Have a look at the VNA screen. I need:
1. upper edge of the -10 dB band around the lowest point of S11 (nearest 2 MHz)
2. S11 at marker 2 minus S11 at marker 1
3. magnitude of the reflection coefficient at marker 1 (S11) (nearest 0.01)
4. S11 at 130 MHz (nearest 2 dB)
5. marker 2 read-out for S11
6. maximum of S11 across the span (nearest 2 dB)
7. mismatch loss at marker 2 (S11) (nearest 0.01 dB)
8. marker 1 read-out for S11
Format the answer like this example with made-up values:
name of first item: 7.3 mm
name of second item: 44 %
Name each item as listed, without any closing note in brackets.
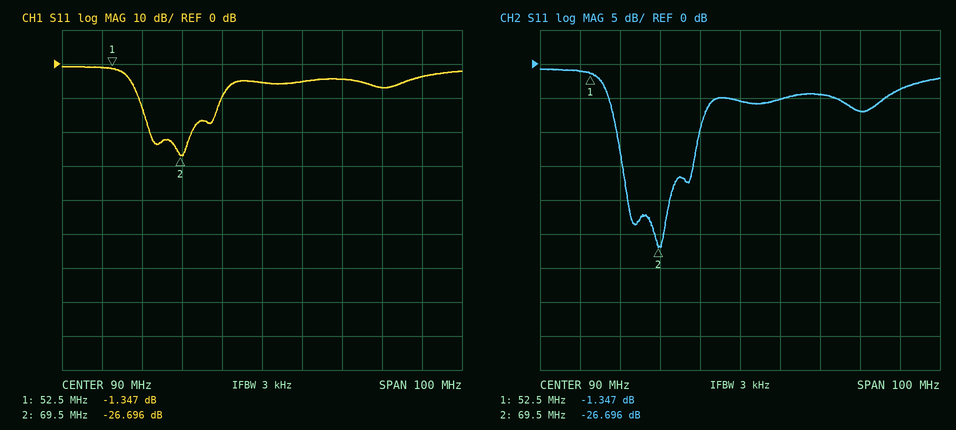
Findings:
upper edge of the -10 dB band around the lowest point of S11: 80 MHz
S11 at marker 2 minus S11 at marker 1: -25.349 dB
magnitude of the reflection coefficient at marker 1 (S11): 0.86
S11 at 130 MHz: -4 dB
marker 2 read-out for S11: -26.696 dB
maximum of S11 across the span: 0 dB
mismatch loss at marker 2 (S11): 0.01 dB
marker 1 read-out for S11: -1.347 dB
